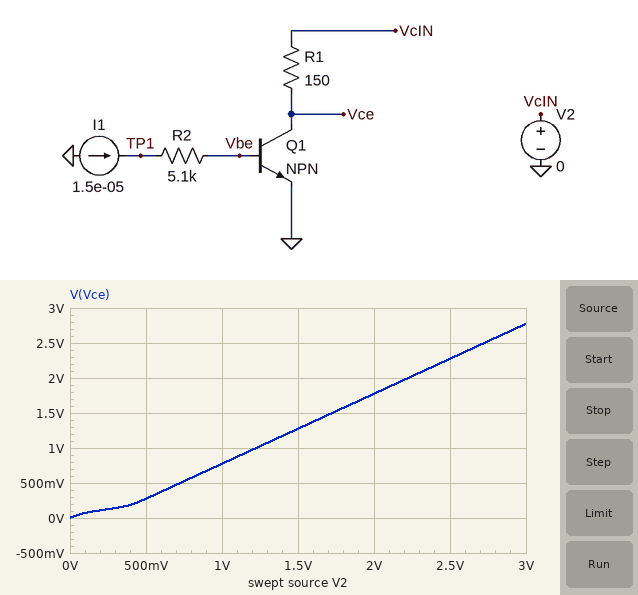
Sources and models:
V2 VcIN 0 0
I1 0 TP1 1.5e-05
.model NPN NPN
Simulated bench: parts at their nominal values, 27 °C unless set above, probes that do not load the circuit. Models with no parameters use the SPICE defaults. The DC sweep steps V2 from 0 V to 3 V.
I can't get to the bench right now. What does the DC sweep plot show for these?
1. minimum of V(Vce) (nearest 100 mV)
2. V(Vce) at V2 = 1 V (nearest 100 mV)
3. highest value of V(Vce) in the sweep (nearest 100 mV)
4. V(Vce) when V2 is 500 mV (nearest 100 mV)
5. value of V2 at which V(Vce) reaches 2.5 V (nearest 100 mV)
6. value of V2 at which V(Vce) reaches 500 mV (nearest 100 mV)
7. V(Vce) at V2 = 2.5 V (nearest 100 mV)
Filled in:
0 V
800 mV
2.8 V
300 mV
2.7 V
700 mV
2.3 V
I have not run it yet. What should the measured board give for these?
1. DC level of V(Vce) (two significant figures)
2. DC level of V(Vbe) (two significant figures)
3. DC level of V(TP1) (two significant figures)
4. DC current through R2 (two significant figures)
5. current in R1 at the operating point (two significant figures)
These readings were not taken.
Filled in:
2.0 mV
670 mV
740 mV
15 µA
14 µA
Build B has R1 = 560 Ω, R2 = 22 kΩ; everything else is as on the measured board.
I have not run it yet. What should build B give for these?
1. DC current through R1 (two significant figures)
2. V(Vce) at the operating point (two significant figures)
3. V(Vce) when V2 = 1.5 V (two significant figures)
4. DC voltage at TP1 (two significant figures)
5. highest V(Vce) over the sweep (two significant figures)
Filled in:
11 µA
6.1 mV
660 mV
1.0 V
2.2 V
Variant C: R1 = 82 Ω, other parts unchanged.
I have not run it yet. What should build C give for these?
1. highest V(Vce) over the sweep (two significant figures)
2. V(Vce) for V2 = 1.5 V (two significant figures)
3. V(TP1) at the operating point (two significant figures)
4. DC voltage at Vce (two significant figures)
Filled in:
2.9 V
1.4 V
740 mV
1.2 mV
